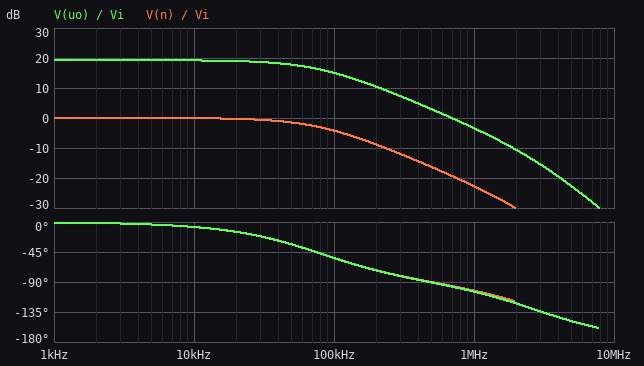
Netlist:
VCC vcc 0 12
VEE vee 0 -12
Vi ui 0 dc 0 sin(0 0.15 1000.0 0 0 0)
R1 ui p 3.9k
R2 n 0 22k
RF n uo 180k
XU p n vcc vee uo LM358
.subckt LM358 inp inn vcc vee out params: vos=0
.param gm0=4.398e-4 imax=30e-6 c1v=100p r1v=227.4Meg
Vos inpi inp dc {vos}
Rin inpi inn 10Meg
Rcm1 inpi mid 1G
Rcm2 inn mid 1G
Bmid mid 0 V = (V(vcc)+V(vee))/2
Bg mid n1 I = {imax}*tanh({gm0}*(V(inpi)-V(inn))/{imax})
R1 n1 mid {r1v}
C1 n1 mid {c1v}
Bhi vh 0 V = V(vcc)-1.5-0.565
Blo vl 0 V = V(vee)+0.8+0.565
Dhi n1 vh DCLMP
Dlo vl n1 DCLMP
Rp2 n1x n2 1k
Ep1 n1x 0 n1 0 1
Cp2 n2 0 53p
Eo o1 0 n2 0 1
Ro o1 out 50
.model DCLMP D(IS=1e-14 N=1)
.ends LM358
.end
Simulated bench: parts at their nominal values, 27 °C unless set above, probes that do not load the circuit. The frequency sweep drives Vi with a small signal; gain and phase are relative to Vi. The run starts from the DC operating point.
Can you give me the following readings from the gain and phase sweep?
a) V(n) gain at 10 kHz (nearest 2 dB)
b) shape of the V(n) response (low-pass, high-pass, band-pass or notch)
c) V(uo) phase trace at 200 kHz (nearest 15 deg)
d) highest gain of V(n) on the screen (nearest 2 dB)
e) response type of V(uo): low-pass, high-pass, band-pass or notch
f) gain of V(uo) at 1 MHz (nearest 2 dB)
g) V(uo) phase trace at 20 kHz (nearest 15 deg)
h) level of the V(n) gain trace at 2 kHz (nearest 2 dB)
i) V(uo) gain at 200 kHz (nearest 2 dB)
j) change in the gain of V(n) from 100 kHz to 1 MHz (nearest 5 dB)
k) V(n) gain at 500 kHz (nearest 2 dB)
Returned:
0 dB
low-pass
-75 deg
0 dB
low-pass
-4 dB
-15 deg
0 dB
10 dB
-20 dB
-16 dB
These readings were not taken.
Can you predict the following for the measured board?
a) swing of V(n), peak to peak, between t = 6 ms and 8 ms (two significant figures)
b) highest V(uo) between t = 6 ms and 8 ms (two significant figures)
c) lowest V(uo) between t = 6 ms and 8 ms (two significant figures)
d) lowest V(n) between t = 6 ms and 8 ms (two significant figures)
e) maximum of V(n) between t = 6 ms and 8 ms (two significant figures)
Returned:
300 mV
1.4 V
-1.4 V
-150 mV
150 mV
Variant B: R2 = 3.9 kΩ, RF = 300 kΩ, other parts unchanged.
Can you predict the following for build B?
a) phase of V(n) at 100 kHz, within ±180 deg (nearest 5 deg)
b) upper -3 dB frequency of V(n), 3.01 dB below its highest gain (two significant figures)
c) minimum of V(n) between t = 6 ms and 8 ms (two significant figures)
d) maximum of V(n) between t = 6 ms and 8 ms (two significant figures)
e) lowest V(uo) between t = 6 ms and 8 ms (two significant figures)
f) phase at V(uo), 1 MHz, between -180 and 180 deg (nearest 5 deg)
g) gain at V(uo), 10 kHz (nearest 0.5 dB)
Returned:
-85 deg
9.0 kHz
-140 mV
130 mV
-11 V
-110 deg
34.5 dB
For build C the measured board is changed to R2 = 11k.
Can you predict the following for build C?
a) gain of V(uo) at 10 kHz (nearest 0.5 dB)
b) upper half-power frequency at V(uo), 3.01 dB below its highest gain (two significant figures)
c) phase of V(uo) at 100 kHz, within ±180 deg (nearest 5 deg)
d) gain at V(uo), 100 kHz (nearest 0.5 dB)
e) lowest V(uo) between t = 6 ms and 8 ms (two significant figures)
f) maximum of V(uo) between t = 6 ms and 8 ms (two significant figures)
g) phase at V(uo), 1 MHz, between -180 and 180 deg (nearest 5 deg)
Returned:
24.5 dB
41 kHz
-70 deg
16.5 dB
-2.6 V
2.6 V
-105 deg
